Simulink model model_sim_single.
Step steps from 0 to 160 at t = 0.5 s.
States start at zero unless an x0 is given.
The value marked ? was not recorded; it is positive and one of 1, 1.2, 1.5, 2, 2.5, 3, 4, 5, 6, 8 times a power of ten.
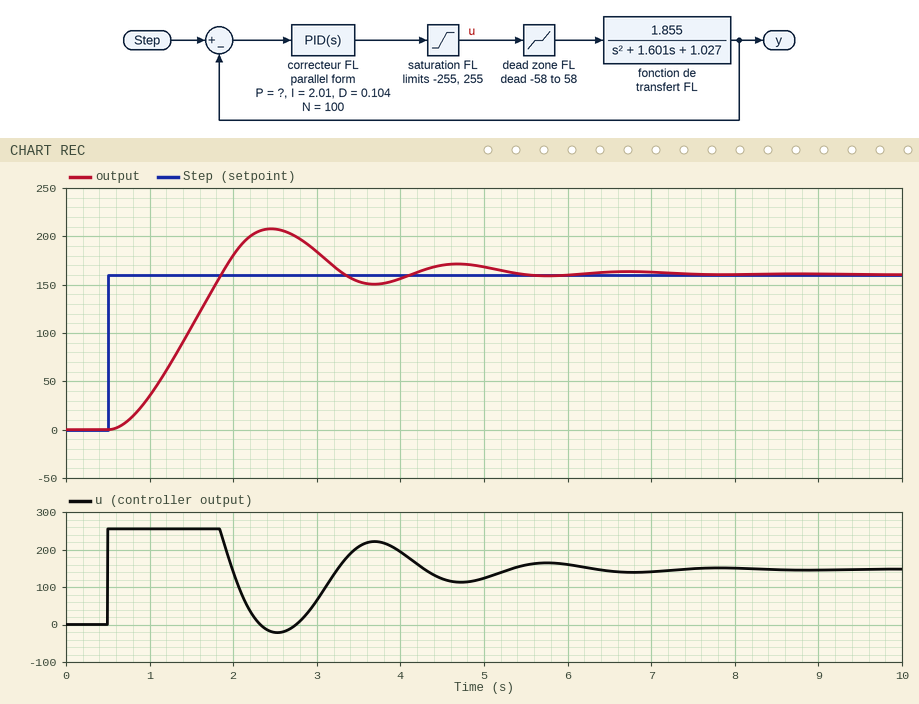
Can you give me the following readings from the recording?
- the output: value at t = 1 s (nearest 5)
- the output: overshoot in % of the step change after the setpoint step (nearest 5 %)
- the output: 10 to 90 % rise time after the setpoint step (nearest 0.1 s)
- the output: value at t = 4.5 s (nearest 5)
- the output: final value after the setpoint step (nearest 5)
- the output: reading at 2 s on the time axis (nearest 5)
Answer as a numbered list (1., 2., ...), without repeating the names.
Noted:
1. 35
2. 30 %
3. 0.9 s
4. 170
5. 160
6. 180
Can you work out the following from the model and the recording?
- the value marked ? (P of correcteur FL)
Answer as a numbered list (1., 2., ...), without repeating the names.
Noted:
1. 5
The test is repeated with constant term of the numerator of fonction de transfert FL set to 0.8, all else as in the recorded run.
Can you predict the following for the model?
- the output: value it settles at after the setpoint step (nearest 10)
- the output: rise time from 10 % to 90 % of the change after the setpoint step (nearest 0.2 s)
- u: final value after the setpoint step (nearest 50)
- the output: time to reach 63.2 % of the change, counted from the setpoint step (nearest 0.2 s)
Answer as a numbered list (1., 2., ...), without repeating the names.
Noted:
1. 150
2. 2.4 s
3. 250
4. 1.8 s
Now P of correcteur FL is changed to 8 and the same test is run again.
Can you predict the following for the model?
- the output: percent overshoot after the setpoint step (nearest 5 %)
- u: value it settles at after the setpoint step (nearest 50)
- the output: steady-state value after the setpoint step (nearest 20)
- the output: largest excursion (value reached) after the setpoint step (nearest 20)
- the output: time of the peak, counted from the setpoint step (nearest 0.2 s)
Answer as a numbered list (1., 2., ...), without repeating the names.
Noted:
1. 25 %
2. 150
3. 160
4. 200
5. 1.8 s
